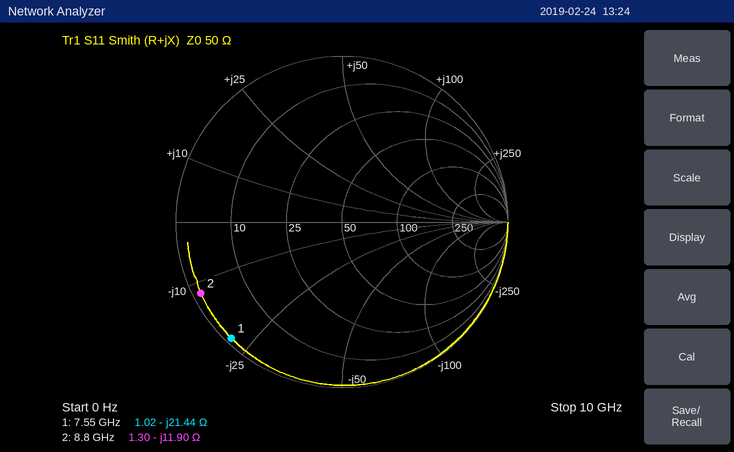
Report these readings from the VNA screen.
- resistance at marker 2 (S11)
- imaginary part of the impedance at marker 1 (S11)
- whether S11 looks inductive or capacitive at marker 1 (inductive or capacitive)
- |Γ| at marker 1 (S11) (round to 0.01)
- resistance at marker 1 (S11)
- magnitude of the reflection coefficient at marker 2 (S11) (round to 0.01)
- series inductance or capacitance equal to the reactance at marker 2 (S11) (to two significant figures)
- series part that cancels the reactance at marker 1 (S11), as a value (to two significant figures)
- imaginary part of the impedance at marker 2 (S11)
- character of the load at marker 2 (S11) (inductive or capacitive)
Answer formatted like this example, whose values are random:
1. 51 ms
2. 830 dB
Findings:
1. 1.30 Ω
2. -21.44 Ω
3. capacitive
4. 0.97
5. 1.02 Ω
6. 0.95
7. 1.5 pF
8. 450 pH
9. -11.90 Ω
10. capacitive
